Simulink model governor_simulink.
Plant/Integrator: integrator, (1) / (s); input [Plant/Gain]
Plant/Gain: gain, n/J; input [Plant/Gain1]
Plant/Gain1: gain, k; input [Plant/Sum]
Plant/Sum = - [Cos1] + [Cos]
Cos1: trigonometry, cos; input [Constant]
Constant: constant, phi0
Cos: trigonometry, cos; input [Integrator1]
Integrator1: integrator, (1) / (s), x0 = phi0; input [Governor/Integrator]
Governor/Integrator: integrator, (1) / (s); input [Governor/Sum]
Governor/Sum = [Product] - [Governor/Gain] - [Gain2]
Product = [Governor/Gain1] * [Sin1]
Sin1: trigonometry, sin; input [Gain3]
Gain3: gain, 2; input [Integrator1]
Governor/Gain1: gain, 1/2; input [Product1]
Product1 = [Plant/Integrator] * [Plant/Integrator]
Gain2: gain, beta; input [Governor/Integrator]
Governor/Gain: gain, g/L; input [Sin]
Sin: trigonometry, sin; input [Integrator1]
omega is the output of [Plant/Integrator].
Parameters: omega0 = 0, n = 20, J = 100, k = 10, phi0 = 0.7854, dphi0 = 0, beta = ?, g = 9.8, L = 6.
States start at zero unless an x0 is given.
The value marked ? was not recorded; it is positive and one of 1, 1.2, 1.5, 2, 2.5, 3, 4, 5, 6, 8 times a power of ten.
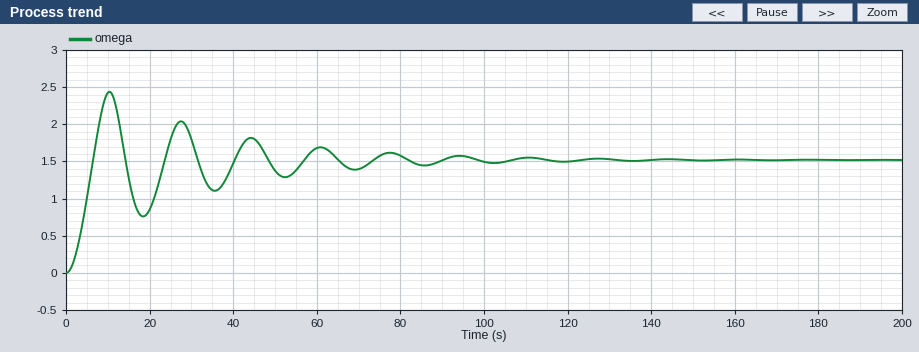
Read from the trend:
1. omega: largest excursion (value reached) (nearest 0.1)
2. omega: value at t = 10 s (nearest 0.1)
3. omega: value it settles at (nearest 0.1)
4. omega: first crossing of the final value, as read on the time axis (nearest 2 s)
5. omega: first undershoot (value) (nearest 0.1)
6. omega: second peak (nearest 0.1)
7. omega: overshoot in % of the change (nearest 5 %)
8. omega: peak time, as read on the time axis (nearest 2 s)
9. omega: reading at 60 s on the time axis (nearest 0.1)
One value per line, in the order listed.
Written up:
2.4
2.4
1.5
6 s
0.8
2.0
60 %
10 s
1.7
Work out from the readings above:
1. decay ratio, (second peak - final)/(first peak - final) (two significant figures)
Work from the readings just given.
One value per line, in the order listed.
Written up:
0.56
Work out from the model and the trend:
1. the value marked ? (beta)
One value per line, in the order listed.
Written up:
15
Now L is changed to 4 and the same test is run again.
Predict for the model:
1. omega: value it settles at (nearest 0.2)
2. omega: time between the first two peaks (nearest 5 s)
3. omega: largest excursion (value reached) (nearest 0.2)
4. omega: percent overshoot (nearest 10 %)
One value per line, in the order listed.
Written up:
1.8
15 s
3.0
60 %
